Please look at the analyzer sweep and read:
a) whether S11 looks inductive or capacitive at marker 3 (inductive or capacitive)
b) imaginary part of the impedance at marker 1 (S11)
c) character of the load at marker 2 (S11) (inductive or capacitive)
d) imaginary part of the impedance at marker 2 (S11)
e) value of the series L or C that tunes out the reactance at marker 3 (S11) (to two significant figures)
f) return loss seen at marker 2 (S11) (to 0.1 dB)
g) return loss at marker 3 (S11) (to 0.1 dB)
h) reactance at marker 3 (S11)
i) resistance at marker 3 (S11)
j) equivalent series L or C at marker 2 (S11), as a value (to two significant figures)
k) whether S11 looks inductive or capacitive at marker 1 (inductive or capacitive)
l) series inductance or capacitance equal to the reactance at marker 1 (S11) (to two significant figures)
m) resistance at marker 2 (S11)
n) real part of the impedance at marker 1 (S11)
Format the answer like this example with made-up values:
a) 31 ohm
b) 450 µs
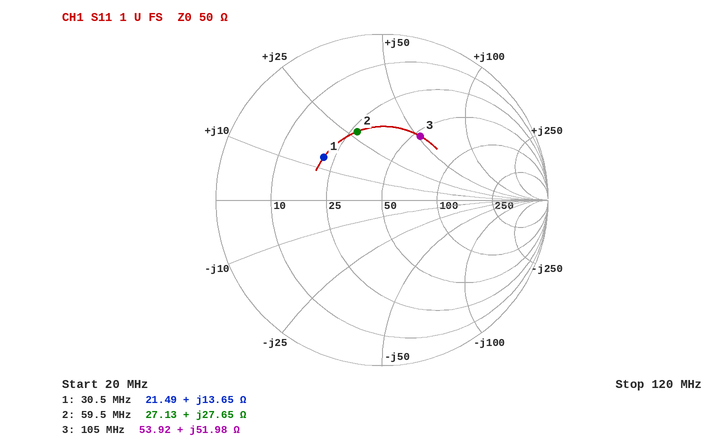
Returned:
a) inductive
b) +13.65 Ω
c) inductive
d) +27.65 Ω
e) 29 pF
f) 7.2 dB
g) 7.0 dB
h) +51.98 Ω
i) 53.92 Ω
j) 74 nH
k) inductive
l) 71 nH
m) 27.13 Ω
n) 21.49 Ω
